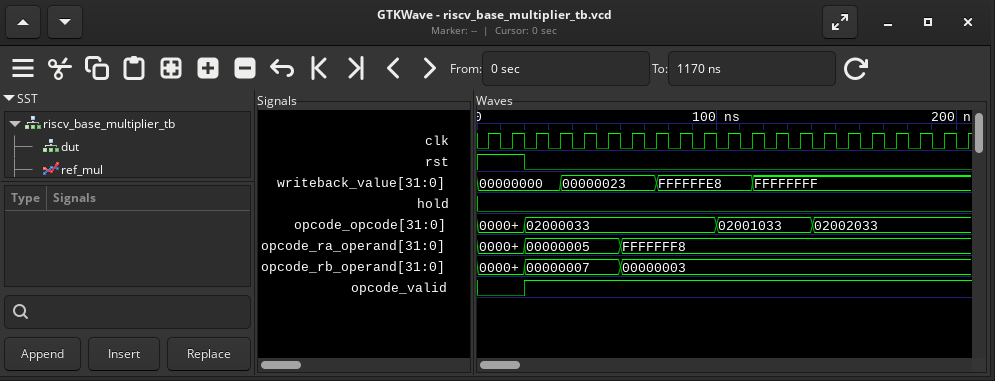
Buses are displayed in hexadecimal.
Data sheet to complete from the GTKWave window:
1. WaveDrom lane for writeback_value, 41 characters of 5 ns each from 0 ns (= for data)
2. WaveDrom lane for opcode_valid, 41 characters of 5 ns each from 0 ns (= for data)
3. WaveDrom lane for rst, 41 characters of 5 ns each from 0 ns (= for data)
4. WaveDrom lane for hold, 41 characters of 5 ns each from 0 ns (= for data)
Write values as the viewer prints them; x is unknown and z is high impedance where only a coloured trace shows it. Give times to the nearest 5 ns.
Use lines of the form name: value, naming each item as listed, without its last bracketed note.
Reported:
WaveDrom lane for writeback_value, 41 characters of 5 ns each from 0 ns: {name: 'writeback_value', wave: '=......=.......=.......=.................', data: '00000000 00000023 FFFFFFE8 FFFFFFFF'}
WaveDrom lane for opcode_valid, 41 characters of 5 ns each from 0 ns: {name: 'opcode_valid', wave: '0...1....................................'}
WaveDrom lane for rst, 41 characters of 5 ns each from 0 ns: {name: 'rst', wave: '1...0....................................'}
WaveDrom lane for hold, 41 characters of 5 ns each from 0 ns: {name: 'hold', wave: '0........................................'}
